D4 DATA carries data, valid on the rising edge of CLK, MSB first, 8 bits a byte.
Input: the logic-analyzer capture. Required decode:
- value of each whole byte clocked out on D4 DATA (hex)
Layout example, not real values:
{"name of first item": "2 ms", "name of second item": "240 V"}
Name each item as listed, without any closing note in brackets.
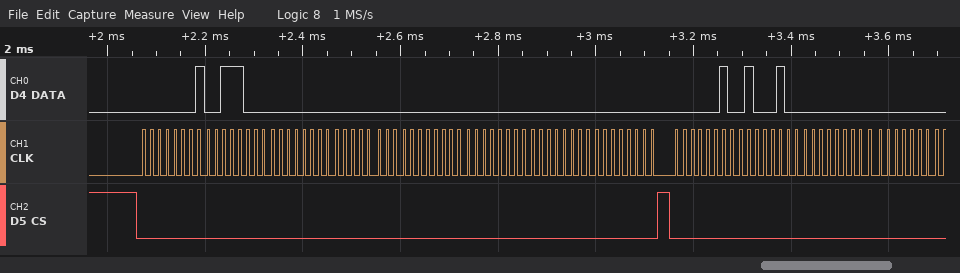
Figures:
{"value of each whole byte clocked out on D4 DATA": "01 38 00 00 00 00 00 00 02 44 00 00"}
